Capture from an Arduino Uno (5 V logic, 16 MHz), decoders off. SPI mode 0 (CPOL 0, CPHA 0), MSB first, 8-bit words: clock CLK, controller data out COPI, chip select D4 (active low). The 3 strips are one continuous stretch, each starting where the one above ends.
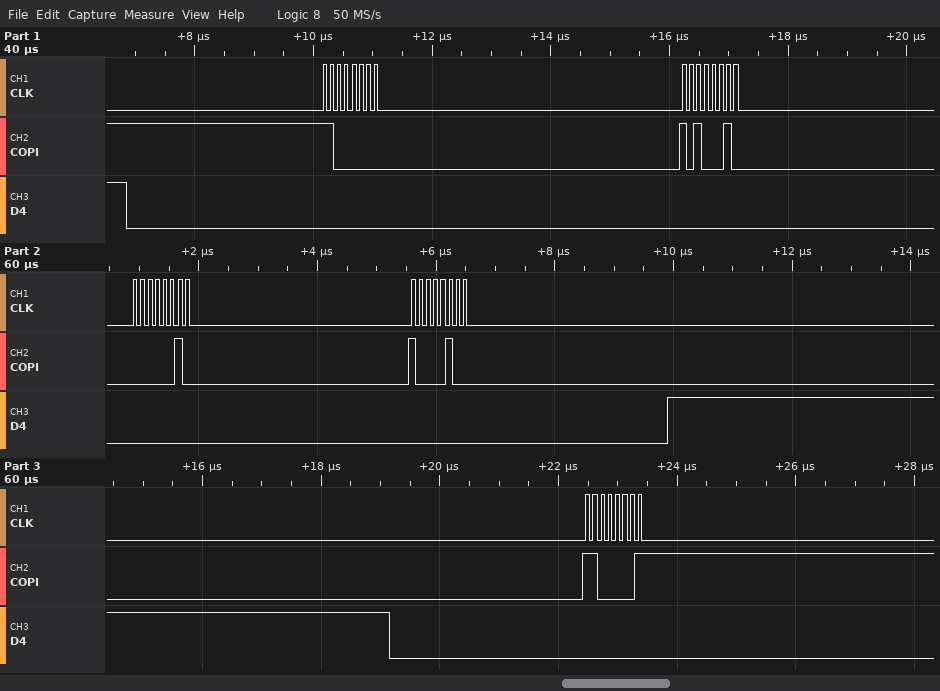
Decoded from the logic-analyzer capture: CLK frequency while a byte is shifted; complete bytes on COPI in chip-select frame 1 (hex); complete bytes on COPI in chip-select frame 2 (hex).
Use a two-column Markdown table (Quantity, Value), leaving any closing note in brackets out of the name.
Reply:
| Quantity | Value |
|---|---|
| CLK frequency while a byte is shifted | 8 MHz |
| complete bytes on COPI in chip-select frame 1 | C0 A2 02 84 |
| complete bytes on COPI in chip-select frame 2 | C1 |
